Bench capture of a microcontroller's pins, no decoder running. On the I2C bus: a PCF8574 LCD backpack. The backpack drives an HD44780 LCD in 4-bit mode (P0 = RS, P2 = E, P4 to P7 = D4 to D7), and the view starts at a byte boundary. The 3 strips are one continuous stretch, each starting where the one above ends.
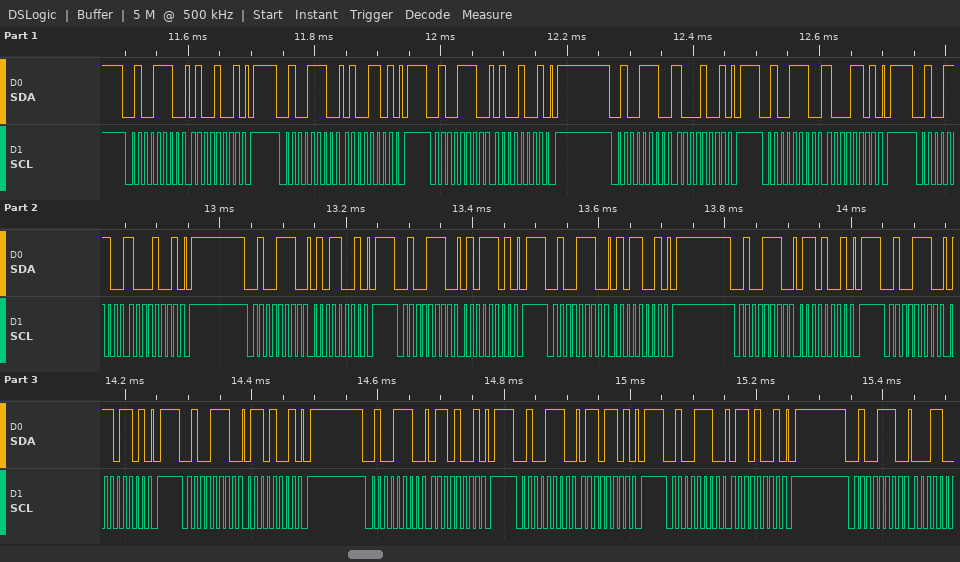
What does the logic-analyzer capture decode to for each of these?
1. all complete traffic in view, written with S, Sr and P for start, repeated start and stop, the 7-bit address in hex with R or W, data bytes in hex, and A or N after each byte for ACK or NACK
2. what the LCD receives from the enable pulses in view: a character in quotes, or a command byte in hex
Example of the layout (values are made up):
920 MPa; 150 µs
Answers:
S 27W A 49 A P S 27W A 4D A P S 27W A 49 A P S 27W A 89 A P S 27W A 8D A P S 27W A 89 A P S 27W A 59 A P S 27W A 5D A P S 27W A 59 A P S 27W A 69 A P S 27W A 6D A P S 27W A 69 A P S 27W A 69 A P S 27W A 6D A P S 27W A 69 A P S 27W A; 'H' 'V'
